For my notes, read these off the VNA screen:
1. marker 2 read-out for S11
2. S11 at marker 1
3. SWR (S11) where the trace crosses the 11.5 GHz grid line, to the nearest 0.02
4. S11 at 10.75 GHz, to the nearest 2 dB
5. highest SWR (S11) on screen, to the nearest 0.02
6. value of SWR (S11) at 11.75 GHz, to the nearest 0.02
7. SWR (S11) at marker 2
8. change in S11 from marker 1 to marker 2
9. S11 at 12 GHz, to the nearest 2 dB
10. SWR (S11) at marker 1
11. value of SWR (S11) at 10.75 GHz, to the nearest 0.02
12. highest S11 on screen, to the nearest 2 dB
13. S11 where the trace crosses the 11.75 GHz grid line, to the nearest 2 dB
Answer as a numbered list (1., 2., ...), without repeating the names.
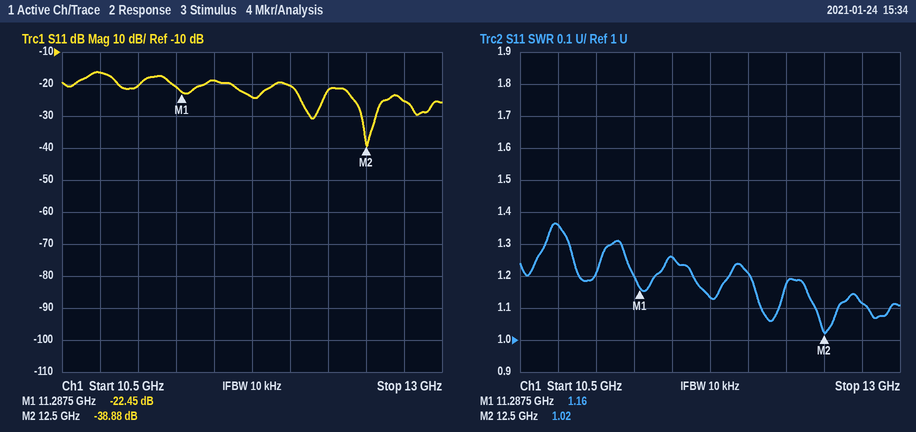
1. -38.88 dB
2. -22.45 dB
3. 1.26
4. -16 dB
5. 1.36
6. 1.14
7. 1.02
8. -16.43 dB
9. -20 dB
10. 1.16
11. 1.36
12. -16 dB
13. -24 dB
